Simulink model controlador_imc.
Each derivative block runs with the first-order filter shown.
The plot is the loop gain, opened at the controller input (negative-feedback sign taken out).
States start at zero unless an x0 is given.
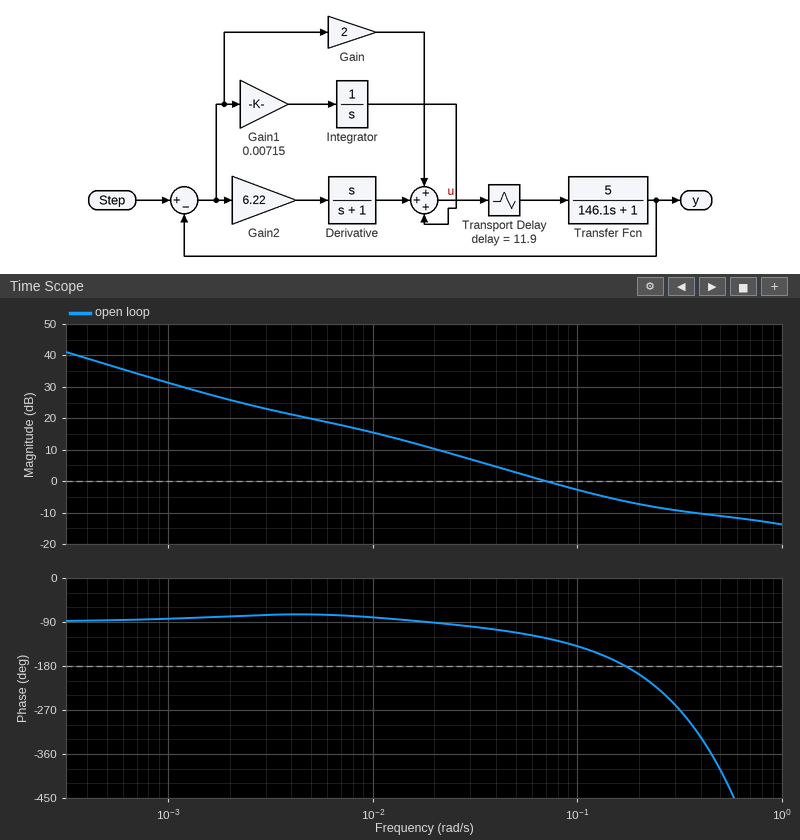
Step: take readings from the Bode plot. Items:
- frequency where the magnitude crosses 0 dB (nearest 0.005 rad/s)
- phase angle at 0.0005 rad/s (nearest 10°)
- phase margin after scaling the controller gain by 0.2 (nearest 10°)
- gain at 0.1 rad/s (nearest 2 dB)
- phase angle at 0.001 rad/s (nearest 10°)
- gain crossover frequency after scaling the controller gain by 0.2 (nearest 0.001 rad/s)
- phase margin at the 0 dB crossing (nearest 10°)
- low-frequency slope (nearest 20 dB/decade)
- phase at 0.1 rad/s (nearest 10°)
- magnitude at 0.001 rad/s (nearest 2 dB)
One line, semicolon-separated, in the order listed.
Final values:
0.070 rad/s; -90°; 100°; -2 dB; -80°; 0.012 rad/s; 60°; -20 dB/decade; -140°; 32 dB
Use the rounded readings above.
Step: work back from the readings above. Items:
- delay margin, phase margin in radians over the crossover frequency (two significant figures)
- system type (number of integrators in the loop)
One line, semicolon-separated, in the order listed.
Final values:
15 s; 1
